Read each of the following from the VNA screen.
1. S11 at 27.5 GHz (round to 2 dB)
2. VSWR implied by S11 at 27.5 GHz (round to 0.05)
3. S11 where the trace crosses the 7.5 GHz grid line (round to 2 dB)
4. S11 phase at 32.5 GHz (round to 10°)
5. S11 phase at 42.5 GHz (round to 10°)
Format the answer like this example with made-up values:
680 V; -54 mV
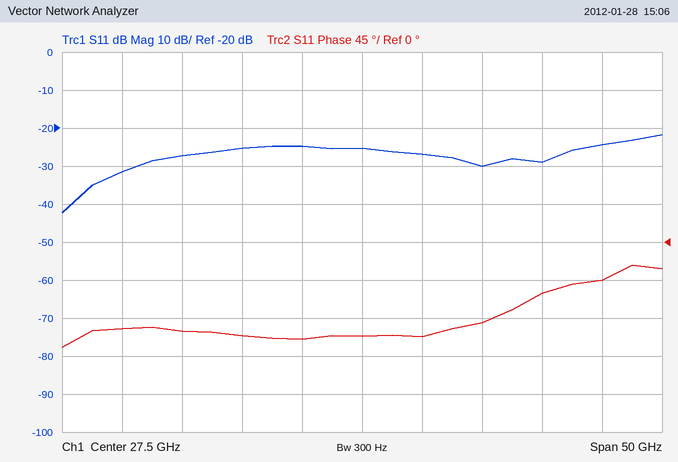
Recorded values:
-26 dB; 1.10; -32 dB; -110°; -60°
